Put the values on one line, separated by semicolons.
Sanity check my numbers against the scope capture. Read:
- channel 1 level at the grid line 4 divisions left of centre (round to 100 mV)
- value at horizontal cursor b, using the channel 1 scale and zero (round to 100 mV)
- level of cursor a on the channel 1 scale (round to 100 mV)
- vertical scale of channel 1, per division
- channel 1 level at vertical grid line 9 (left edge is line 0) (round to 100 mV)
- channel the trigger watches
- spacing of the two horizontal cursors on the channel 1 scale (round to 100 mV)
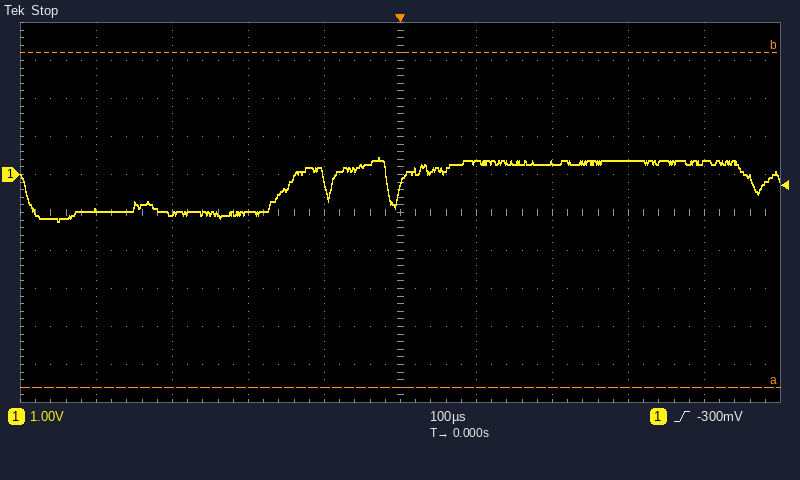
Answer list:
-900 mV; 3.2 V; -5.6 V; 1 V; 300 mV; channel 1; 8.8 V
